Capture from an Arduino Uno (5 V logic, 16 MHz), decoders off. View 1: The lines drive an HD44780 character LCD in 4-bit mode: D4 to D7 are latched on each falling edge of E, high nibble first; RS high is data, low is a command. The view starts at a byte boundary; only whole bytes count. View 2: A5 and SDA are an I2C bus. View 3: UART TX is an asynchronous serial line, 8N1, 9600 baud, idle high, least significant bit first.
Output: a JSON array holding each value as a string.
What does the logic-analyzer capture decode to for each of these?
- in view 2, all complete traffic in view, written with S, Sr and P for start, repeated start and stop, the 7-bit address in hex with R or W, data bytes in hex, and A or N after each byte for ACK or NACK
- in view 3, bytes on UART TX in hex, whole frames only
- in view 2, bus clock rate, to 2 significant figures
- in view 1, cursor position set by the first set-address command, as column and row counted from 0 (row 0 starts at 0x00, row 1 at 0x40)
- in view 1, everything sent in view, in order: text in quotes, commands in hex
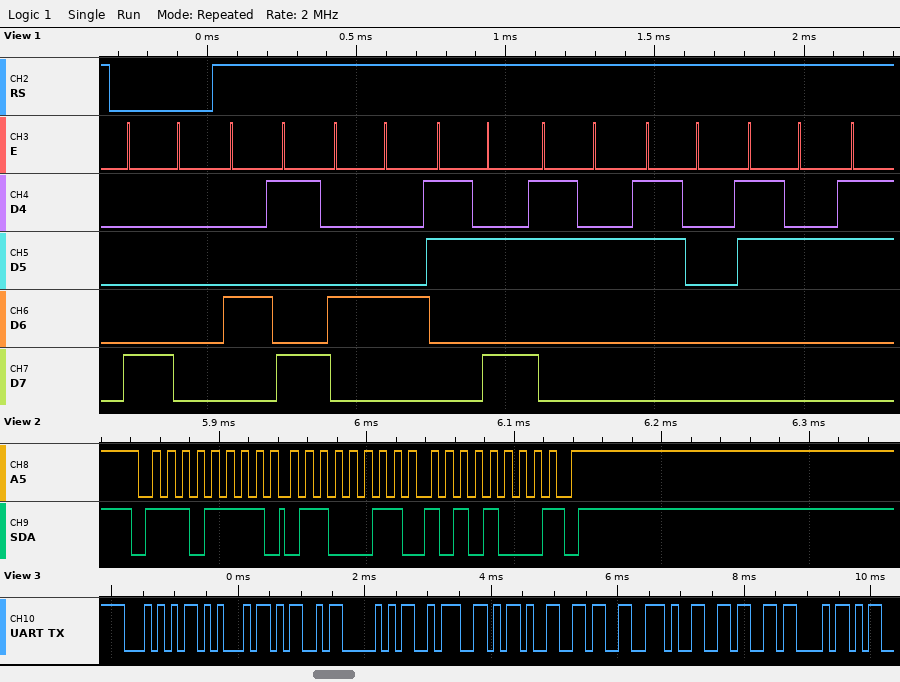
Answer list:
["S 77R A 63 A A8 N P", "54 45 4D 50 3A 2D 36 2E 36 43", "100 kHz", "column 0, row 0", "0x80 \"ID:202\""]
